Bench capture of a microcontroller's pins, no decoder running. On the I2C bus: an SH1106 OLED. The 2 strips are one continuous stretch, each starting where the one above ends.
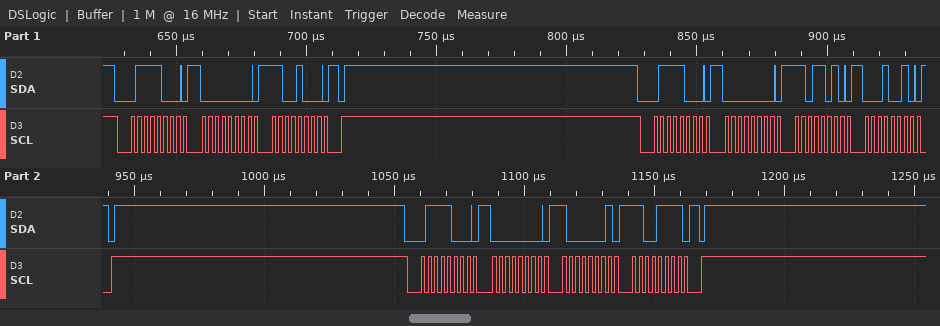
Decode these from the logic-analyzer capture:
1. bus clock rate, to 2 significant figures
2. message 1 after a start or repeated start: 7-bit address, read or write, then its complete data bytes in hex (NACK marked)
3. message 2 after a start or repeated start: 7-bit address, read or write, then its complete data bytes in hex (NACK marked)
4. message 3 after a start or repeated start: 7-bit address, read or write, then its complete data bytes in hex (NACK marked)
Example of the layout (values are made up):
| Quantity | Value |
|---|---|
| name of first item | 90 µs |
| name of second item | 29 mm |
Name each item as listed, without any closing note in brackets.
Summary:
| Quantity | Value |
|---|---|
| bus clock rate, to 2 significant figures | 400 kHz |
| message 1 after a start or repeated start: 7-bit address, read or write, then its complete data bytes in hex | 0x3C write: 00 C8 |
| message 2 after a start or repeated start: 7-bit address, read or write, then its complete data bytes in hex | 0x3C write: 00 DA 12 |
| message 3 after a start or repeated start: 7-bit address, read or write, then its complete data bytes in hex | 0x3C write: 00 81 CF |
